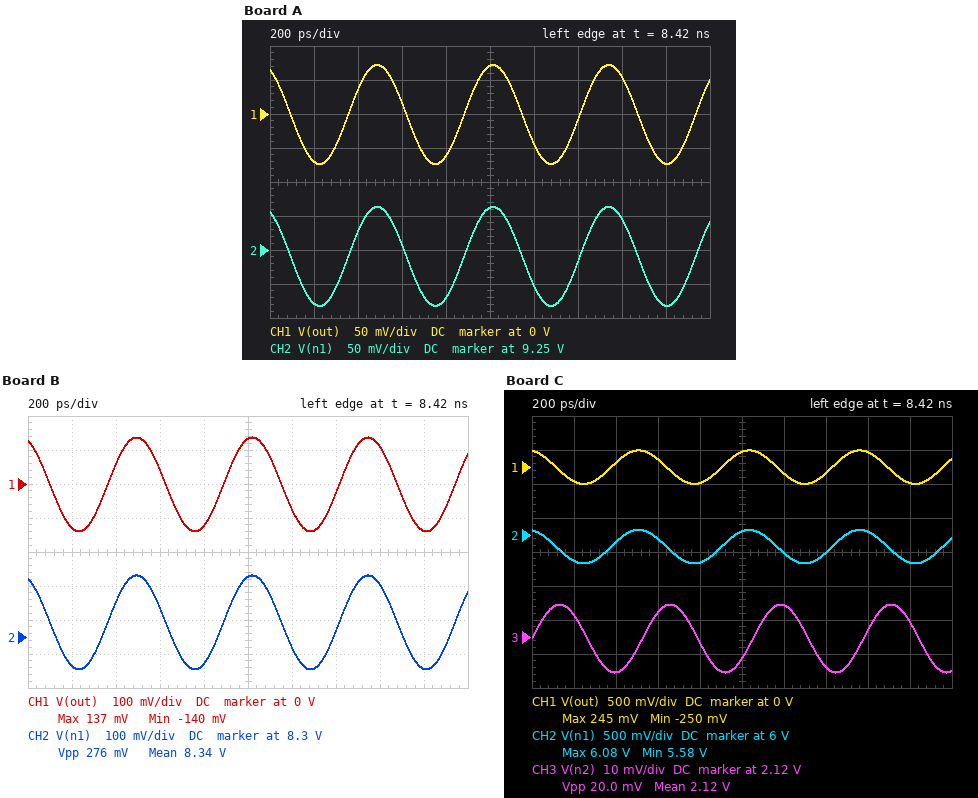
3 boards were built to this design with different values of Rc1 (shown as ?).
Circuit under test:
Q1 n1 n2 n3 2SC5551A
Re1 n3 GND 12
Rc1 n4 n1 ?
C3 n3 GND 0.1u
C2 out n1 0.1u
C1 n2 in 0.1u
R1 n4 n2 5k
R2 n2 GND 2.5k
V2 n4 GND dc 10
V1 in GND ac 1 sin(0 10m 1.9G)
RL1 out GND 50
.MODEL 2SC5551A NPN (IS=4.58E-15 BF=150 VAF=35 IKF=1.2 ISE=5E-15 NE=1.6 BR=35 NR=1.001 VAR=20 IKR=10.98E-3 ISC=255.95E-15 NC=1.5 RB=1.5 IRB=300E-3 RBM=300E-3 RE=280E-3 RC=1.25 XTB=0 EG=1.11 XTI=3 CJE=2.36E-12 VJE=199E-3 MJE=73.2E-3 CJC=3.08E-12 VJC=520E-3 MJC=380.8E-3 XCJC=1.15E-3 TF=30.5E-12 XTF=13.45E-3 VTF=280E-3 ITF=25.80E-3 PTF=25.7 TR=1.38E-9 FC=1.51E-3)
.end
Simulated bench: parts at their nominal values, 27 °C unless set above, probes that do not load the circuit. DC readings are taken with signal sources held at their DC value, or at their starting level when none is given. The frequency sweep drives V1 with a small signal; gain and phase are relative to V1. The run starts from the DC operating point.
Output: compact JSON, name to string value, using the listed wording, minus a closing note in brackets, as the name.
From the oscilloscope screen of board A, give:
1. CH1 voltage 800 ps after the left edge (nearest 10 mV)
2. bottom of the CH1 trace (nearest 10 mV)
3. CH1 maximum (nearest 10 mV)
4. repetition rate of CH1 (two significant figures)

{"CH1 voltage 800 ps after the left edge": "-60 mV", "bottom of the CH1 trace": "-70 mV", "CH1 maximum": "70 mV", "repetition rate of CH1": "1.9 GHz"}
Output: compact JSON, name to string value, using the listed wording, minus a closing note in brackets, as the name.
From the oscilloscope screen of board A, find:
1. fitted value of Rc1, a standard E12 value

{"fitted value of Rc1, a standard E12 value": "6.8 Ω"}
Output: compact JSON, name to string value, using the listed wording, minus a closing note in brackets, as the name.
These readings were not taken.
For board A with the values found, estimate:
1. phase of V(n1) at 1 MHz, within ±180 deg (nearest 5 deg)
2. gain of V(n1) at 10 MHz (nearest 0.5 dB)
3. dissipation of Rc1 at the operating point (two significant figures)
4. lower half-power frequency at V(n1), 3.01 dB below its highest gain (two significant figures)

{"phase of V(n1) at 1 MHz, within ±180 deg": "-115 deg", "gain of V(n1) at 10 MHz": "20.5 dB", "dissipation of Rc1 at the operating point": "85 mW", "lower half-power frequency at V(n1), 3.01 dB below its highest gain": "3.1 MHz"}
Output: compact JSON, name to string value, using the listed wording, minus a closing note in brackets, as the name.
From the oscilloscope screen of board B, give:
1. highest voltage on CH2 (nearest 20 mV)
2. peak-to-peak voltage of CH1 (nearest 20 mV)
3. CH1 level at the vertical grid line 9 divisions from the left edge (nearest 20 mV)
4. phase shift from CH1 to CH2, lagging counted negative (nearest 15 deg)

{"highest voltage on CH2": "8.48 V", "peak-to-peak voltage of CH1": "280 mV", "CH1 level at the vertical grid line 9 divisions from the left edge": "-140 mV", "phase shift from CH1 to CH2, lagging counted negative": "0 deg"}
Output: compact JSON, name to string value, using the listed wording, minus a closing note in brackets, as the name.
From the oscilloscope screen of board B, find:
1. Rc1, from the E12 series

{"Rc1, from the E12 series": "15 Ω"}
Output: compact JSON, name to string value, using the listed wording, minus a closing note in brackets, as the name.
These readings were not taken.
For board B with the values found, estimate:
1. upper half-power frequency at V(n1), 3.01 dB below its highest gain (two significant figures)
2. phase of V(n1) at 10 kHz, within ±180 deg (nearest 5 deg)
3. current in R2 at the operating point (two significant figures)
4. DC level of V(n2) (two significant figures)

{"upper half-power frequency at V(n1), 3.01 dB below its highest gain": "1.7 GHz", "phase of V(n1) at 10 kHz, within ±180 deg": "-170 deg", "current in R2 at the operating point": "860 µA", "DC level of V(n2)": "2.2 V"}
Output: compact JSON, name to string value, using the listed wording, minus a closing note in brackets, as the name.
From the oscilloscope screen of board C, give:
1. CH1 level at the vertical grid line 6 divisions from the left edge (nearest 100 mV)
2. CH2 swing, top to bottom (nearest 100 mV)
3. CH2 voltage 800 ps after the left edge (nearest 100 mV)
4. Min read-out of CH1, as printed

{"CH1 level at the vertical grid line 6 divisions from the left edge": "-100 mV", "CH2 swing, top to bottom": "500 mV", "CH2 voltage 800 ps after the left edge": "5.6 V", "Min read-out of CH1, as printed": "-250 mV"}
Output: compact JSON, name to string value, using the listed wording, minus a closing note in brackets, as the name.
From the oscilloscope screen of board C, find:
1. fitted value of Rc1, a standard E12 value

{"fitted value of Rc1, a standard E12 value": "39 Ω"}
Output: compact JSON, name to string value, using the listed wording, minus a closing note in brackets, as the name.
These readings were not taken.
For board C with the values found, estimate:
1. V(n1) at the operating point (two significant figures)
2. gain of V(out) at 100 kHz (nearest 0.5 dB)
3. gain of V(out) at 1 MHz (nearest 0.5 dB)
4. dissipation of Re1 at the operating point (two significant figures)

{"V(n1) at the operating point": "5.8 V", "gain of V(out) at 100 kHz": "6.5 dB", "gain of V(out) at 1 MHz": "22.0 dB", "dissipation of Re1 at the operating point": "140 mW"}
